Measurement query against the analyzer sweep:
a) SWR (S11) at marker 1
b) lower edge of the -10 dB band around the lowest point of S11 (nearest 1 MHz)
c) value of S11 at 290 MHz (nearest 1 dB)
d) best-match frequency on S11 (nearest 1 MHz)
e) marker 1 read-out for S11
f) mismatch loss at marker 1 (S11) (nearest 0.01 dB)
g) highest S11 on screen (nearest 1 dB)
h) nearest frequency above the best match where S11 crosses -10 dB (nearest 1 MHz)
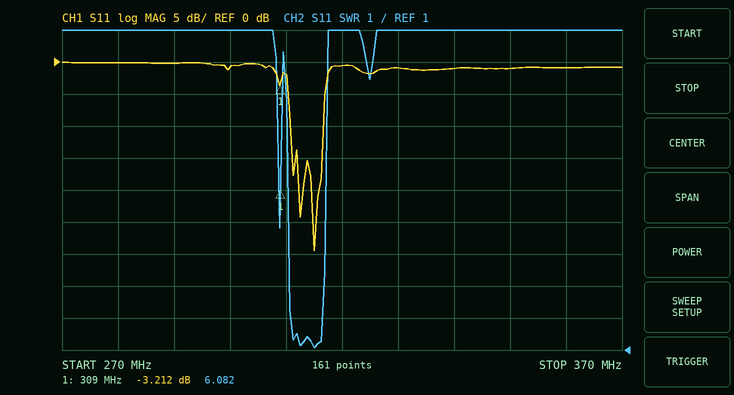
6.082
311 MHz
0 dB
315 MHz
-3.212 dB
2.82 dB
0 dB
317 MHz
